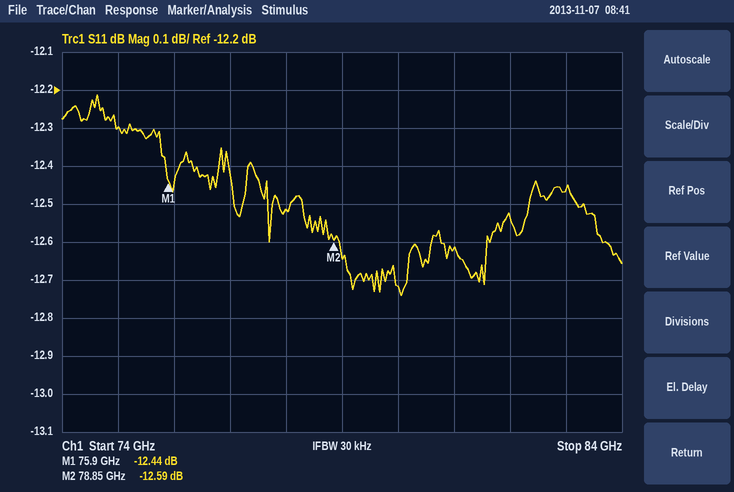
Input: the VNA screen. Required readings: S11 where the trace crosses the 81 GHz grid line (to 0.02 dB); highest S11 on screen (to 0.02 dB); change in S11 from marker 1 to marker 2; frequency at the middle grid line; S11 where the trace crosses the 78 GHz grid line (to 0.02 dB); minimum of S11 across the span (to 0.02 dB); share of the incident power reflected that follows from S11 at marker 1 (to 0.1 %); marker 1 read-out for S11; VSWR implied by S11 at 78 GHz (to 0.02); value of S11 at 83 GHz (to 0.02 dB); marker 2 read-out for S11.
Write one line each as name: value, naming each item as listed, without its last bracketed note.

S11 where the trace crosses the 81 GHz grid line: -12.62 dB
highest S11 on screen: -12.22 dB
change in S11 from marker 1 to marker 2: -0.15 dB
frequency at the middle grid line: 79 GHz
S11 where the trace crosses the 78 GHz grid line: -12.52 dB
minimum of S11 across the span: -12.74 dB
share of the incident power reflected that follows from S11 at marker 1: 5.7 %
marker 1 read-out for S11: -12.44 dB
VSWR implied by S11 at 78 GHz: 1.62
value of S11 at 83 GHz: -12.46 dB
marker 2 read-out for S11: -12.59 dB
